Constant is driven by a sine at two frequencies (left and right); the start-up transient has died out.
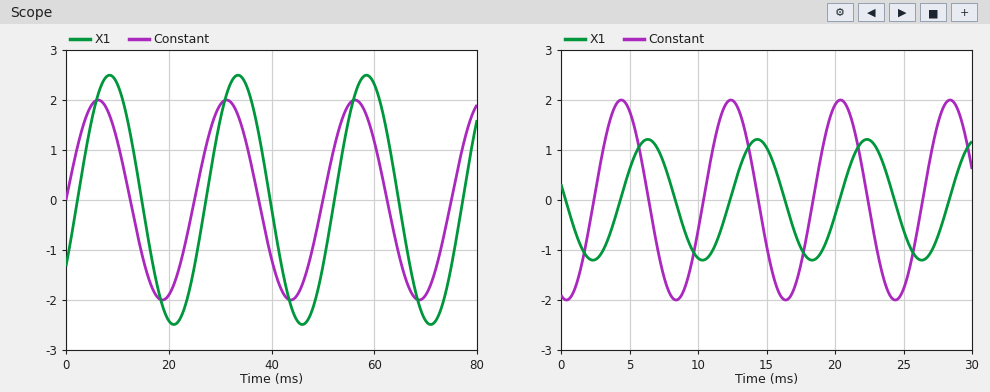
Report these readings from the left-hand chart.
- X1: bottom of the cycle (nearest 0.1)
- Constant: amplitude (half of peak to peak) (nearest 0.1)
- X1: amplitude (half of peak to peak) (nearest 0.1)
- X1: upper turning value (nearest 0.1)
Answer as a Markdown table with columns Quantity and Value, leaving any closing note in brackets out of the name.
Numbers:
| Quantity | Value |
|---|---|
| X1: bottom of the cycle | -2.5 |
| Constant: amplitude (half of peak to peak) | 2.0 |
| X1: amplitude (half of peak to peak) | 2.5 |
| X1: upper turning value | 2.5 |
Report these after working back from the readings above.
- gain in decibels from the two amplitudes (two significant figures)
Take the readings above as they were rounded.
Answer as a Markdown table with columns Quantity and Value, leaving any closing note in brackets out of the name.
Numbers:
| Quantity | Value |
|---|---|
| gain in decibels from the two amplitudes | 1.9 dB |
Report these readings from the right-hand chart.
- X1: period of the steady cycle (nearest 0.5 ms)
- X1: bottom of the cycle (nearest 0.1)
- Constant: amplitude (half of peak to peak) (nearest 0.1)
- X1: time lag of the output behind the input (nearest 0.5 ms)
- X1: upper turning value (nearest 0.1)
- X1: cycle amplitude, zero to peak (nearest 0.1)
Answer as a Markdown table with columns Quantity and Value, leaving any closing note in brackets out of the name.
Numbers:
| Quantity | Value |
|---|---|
| X1: period of the steady cycle | 8.0 ms |
| X1: bottom of the cycle | -1.2 |
| Constant: amplitude (half of peak to peak) | 2.0 |
| X1: time lag of the output behind the input | 2.0 ms |
| X1: upper turning value | 1.2 |
| X1: cycle amplitude, zero to peak | 1.2 |
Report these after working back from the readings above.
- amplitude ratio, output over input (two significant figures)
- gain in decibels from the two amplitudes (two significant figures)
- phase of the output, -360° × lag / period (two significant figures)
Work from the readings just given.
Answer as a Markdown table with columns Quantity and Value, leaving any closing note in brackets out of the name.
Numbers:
| Quantity | Value |
|---|---|
| amplitude ratio, output over input | 0.60 |
| gain in decibels from the two amplitudes | -4.4 dB |
| phase of the output, -360° × lag / period | -90° |
